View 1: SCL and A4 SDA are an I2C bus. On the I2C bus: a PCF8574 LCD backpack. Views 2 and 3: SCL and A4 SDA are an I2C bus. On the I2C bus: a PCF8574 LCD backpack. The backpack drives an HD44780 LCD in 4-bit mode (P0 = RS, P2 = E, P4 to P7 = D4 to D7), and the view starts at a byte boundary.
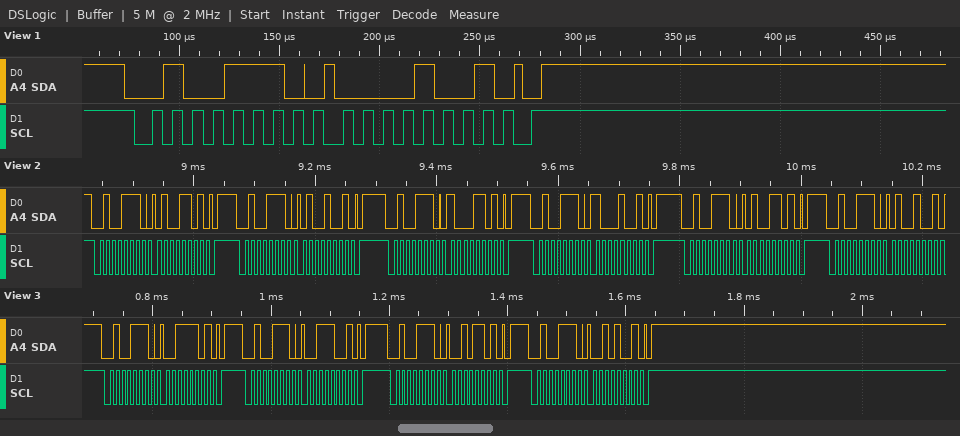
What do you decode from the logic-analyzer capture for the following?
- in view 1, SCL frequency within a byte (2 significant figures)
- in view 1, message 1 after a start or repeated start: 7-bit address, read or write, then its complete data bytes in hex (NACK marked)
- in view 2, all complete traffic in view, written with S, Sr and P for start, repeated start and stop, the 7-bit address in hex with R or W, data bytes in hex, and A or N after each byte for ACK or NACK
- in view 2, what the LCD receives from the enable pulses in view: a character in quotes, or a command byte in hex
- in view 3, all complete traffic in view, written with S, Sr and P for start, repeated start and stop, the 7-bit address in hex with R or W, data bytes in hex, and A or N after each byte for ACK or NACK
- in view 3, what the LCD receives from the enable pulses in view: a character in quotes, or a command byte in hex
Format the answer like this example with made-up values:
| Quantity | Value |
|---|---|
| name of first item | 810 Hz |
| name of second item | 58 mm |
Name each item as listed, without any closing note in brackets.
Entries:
| Quantity | Value |
|---|---|
| in view 1, SCL frequency within a byte | 100 kHz |
| in view 1, message 1 after a start or repeated start: 7-bit address, read or write, then its complete data bytes in hex | 0x27 write: 09 |
| in view 2, all complete traffic in view, written with S, Sr and P for start, repeated start and stop, the 7-bit address in hex with R or W, data bytes in hex, and A or N after each byte for ACK or NACK | S 27W A 4D A P S 27W A 49 A P S 27W A 8D A P S 27W A 89 A P S 27W A 4D A P S 27W A 49 A |
| in view 2, what the LCD receives from the enable pulses in view: a character in quotes, or a command byte in hex | 'H' |
| in view 3, all complete traffic in view, written with S, Sr and P for start, repeated start and stop, the 7-bit address in hex with R or W, data bytes in hex, and A or N after each byte for ACK or NACK | S 27W A 3D A P S 27W A 39 A P S 27W A 2D A P S 27W A 29 A P |
| in view 3, what the LCD receives from the enable pulses in view: a character in quotes, or a command byte in hex | '2' |
